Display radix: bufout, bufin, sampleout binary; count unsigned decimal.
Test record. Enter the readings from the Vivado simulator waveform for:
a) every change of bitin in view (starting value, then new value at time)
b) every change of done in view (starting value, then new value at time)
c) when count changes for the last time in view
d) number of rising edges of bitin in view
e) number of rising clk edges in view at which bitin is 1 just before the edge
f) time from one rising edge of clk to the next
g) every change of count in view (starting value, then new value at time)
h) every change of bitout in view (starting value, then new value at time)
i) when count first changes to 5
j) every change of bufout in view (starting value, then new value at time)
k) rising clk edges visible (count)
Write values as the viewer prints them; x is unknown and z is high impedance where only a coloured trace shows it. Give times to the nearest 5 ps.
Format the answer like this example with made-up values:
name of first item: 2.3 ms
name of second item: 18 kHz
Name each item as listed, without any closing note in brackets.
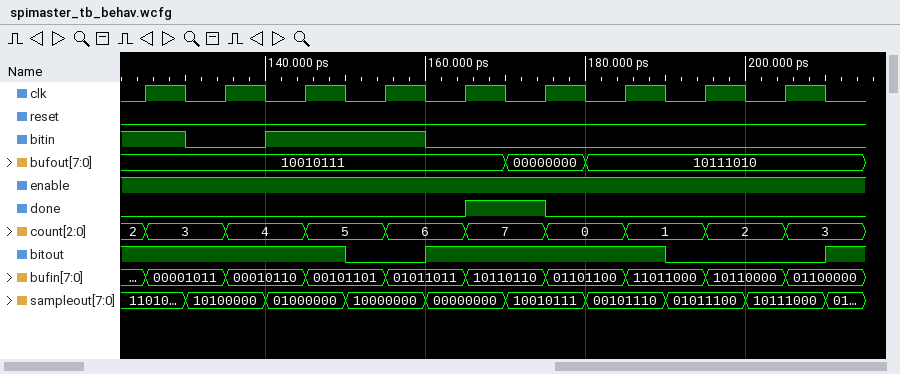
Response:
every change of bitin in view: 1, 0 at 130 ps, 1 at 140 ps, 0 at 160 ps
every change of done in view: 0, 1 at 165 ps, 0 at 175 ps
when count changes for the last time in view: 205 ps
number of rising edges of bitin in view: 1
number of rising clk edges in view at which bitin is 1 just before the edge: 3
time from one rising edge of clk to the next: 10 ps
every change of count in view: 2, 3 at 125 ps, 4 at 135 ps, 5 at 145 ps, 6 at 155 ps, 7 at 165 ps, 0 at 175 ps, 1 at 185 ps, 2 at 195 ps, 3 at 205 ps
every change of bitout in view: 1, 0 at 150 ps, 1 at 160 ps, 0 at 190 ps, 1 at 210 ps
when count first changes to 5: 145 ps
every change of bufout in view: 10010111, 00000000 at 170 ps, 10111010 at 180 ps
rising clk edges visible: 9
